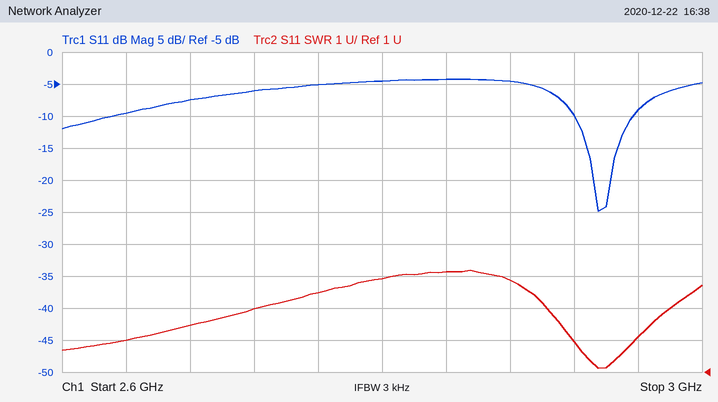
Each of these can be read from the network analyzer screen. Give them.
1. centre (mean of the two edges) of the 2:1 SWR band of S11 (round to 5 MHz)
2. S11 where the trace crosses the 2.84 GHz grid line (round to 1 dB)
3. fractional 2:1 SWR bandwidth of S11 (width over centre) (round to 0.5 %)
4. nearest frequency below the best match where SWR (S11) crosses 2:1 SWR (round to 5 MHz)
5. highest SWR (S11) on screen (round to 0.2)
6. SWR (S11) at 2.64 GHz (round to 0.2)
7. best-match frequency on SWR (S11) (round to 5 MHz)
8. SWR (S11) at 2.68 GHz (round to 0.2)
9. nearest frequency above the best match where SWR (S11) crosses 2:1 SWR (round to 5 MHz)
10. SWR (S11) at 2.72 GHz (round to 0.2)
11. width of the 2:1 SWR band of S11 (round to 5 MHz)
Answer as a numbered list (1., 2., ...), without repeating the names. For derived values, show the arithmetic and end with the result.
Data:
1. 2.940 GHz
2. -4 dB
3. 40 MHz / 2.94 GHz ≈ 1.36 %, so 1.5 % to the nearest 0.5 %
4. 2.920 GHz
5. 4.2
6. 2.0
7. 2.935 GHz
8. 2.4
9. 2.960 GHz
10. 3.0
11. 2.960 GHz − 2.920 GHz = 40 MHz
